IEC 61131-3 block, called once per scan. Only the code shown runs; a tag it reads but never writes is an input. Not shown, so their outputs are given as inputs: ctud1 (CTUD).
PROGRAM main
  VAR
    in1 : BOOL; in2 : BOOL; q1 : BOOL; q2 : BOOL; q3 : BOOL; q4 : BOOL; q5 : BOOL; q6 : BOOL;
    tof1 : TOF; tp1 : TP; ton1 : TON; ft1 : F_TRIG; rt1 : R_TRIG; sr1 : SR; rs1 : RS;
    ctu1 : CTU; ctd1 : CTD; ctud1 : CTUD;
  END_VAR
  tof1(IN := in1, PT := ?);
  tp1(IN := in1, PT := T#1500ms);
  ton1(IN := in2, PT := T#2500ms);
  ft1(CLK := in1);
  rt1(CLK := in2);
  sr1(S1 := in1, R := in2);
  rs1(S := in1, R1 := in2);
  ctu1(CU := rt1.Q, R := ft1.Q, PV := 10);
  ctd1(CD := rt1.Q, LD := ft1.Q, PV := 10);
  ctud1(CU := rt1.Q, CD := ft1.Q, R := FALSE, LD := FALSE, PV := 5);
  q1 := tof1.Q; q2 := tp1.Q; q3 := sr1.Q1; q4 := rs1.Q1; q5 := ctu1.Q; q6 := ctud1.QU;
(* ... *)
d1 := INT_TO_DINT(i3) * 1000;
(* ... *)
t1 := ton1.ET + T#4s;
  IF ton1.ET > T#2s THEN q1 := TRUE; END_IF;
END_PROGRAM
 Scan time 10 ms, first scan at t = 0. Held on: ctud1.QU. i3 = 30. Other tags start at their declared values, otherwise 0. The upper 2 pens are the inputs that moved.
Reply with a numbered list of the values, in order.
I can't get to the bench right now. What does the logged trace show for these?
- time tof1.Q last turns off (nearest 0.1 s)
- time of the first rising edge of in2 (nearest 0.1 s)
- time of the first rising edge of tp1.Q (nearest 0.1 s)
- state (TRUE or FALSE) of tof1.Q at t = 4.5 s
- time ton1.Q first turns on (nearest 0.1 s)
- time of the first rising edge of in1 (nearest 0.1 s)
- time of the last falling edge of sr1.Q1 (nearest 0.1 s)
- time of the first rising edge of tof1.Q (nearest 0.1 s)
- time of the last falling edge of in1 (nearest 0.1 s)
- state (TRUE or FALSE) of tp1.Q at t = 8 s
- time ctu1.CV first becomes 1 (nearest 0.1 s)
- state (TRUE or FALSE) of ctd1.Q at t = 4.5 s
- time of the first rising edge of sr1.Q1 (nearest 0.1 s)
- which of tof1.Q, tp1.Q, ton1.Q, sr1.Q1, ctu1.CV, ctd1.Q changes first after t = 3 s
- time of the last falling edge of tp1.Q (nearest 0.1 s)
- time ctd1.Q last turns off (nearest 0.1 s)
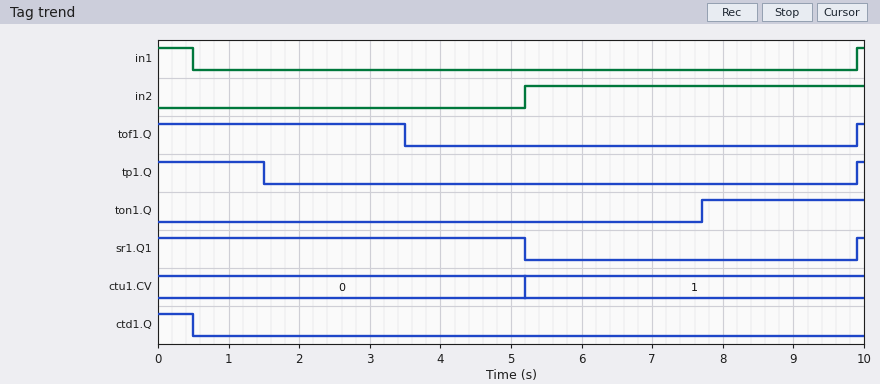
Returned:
1. 3.5 s
2. 5.2 s
3. 9.9 s
4. FALSE
5. 7.7 s
6. 9.9 s
7. 5.2 s
8. 9.9 s
9. 0.5 s
10. FALSE
11. 5.2 s
12. FALSE
13. 9.9 s
14. tof1.Q
15. 1.5 s
16. 0.5 s
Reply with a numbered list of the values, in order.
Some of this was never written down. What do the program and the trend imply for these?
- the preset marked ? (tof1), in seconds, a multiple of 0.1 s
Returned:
1. 3.0 s
